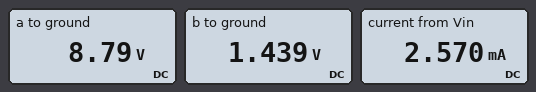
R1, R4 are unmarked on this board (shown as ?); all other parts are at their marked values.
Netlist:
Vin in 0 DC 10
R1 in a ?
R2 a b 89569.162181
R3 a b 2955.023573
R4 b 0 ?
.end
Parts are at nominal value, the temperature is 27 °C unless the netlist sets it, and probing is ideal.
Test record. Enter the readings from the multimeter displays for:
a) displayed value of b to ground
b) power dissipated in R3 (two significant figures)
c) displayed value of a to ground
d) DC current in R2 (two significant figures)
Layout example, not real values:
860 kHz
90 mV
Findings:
1.439 V
18 mW
8.79 V
82 µA
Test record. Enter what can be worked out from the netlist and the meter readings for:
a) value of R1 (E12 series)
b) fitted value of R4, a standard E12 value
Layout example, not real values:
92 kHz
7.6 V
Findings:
470 Ω
560 Ω
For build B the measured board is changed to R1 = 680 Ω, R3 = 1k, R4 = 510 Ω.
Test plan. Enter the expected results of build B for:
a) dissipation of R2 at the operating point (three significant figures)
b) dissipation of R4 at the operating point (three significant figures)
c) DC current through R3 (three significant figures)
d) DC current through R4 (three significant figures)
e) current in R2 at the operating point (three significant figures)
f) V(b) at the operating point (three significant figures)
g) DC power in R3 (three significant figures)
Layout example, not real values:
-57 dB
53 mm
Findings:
230 µW
10.7 mW
4.54 mA
4.59 mA
50.7 µA
2.34 V
20.6 mW
